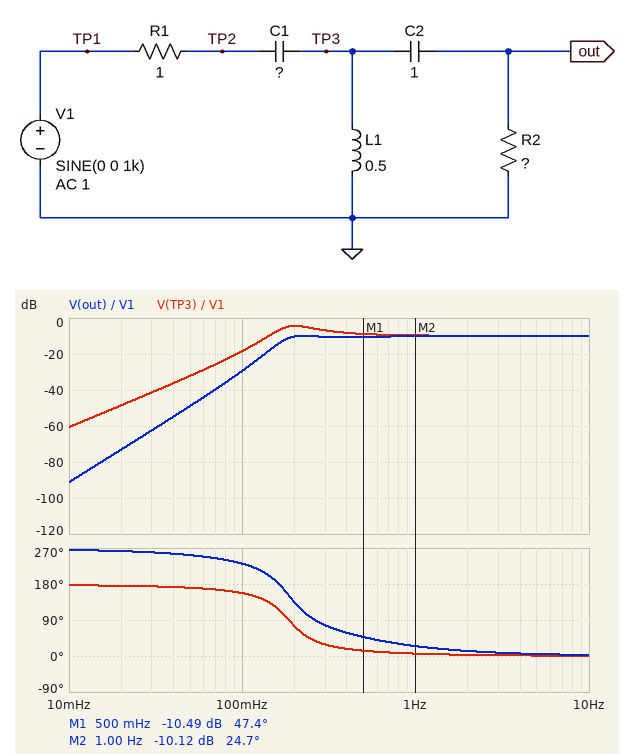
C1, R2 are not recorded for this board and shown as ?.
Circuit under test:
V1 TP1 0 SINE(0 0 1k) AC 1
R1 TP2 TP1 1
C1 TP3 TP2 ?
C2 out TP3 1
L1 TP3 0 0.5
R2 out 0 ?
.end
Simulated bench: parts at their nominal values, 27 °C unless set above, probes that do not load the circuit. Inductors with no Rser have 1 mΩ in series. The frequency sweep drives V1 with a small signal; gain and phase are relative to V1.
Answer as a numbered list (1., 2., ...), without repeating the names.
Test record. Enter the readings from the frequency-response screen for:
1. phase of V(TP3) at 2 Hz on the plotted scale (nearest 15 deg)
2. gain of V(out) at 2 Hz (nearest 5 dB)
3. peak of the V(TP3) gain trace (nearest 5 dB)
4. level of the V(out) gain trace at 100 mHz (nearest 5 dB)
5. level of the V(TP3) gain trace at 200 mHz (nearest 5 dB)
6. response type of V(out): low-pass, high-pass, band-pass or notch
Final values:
1. 0 deg
2. -10 dB
3. -5 dB
4. -30 dB
5. -5 dB
6. high-pass
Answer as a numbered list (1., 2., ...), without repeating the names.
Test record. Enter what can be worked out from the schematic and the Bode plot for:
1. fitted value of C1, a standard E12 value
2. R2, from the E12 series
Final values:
1. 470 mF
2. 0.47 Ω
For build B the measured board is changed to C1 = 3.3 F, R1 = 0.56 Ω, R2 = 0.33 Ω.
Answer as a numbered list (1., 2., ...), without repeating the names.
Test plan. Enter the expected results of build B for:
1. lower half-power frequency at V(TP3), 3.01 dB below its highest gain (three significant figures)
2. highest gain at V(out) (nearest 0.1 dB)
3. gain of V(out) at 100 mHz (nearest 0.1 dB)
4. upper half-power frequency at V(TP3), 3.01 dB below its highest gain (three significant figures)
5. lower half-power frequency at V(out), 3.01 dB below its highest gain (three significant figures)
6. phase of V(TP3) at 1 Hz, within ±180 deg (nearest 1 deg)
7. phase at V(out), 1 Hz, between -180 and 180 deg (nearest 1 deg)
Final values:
1. 99.1 mHz
2. -8.6 dB
3. -17.5 dB
4. 306 mHz
5. 144 mHz
6. -9 deg
7. 17 deg
